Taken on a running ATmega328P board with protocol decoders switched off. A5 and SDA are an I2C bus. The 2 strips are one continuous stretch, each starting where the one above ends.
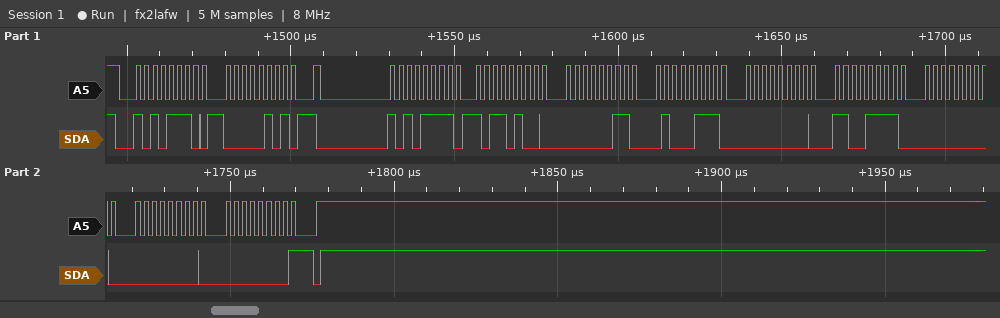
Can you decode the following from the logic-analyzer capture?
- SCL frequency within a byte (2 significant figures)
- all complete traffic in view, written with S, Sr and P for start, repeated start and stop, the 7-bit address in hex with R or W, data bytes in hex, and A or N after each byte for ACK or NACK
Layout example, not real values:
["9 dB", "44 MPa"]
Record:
["400 kHz", "S 57W A 05 A Sr 57R A B4 A 03 A 47 A 00 A CF A 00 A 00 A 00 N P"]
